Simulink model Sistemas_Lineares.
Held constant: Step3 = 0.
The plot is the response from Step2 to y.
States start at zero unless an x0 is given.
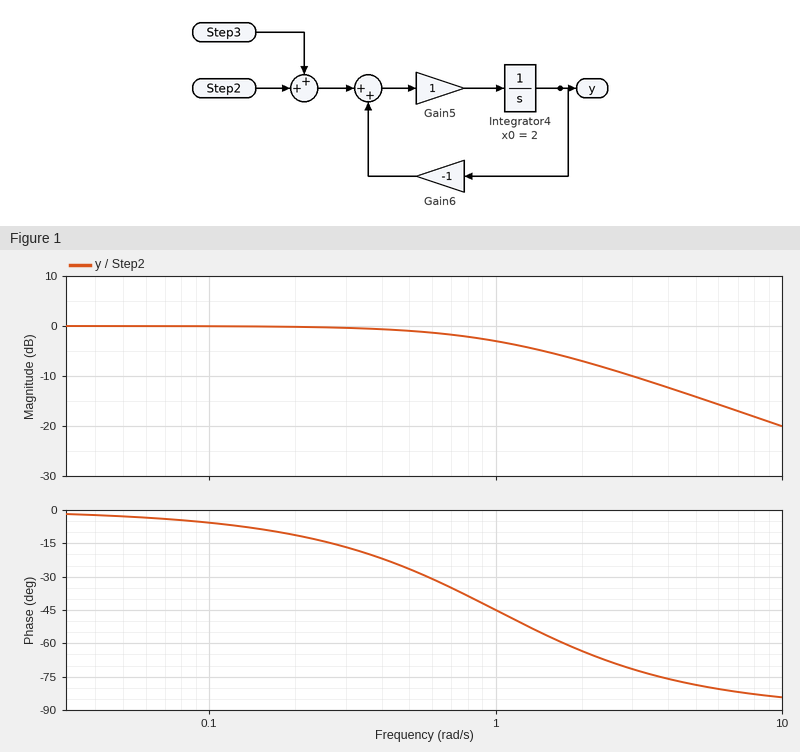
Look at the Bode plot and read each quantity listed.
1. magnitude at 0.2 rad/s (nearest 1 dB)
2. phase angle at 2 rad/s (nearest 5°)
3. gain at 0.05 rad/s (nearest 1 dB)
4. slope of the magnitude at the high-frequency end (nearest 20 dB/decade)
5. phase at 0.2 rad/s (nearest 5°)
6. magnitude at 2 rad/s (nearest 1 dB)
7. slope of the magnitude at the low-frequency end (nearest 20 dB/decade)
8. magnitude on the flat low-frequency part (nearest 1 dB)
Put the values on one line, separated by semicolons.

0 dB; -65°; 0 dB; -20 dB/decade; -10°; -7 dB; 0 dB/decade; 0 dB
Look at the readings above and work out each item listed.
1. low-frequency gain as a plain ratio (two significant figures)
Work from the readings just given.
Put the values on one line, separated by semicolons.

1.0
